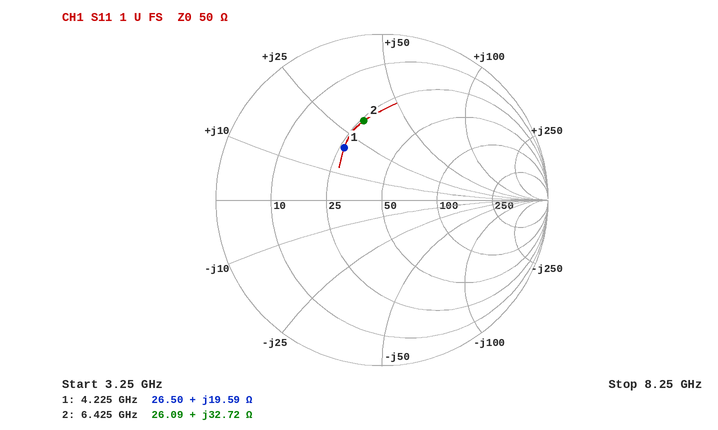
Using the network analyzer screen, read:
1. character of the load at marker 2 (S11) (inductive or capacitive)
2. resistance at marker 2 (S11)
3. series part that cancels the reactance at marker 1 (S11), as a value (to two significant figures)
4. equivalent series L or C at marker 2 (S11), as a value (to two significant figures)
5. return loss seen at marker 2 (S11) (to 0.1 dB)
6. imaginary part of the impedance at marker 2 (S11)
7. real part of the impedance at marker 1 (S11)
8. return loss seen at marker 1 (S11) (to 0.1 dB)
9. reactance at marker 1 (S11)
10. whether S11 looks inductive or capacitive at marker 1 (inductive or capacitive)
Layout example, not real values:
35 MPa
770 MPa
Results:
inductive
26.09 Ω
1.9 pF
810 pH
6.2 dB
+32.72 Ω
26.50 Ω
8.2 dB
+19.59 Ω
inductive
